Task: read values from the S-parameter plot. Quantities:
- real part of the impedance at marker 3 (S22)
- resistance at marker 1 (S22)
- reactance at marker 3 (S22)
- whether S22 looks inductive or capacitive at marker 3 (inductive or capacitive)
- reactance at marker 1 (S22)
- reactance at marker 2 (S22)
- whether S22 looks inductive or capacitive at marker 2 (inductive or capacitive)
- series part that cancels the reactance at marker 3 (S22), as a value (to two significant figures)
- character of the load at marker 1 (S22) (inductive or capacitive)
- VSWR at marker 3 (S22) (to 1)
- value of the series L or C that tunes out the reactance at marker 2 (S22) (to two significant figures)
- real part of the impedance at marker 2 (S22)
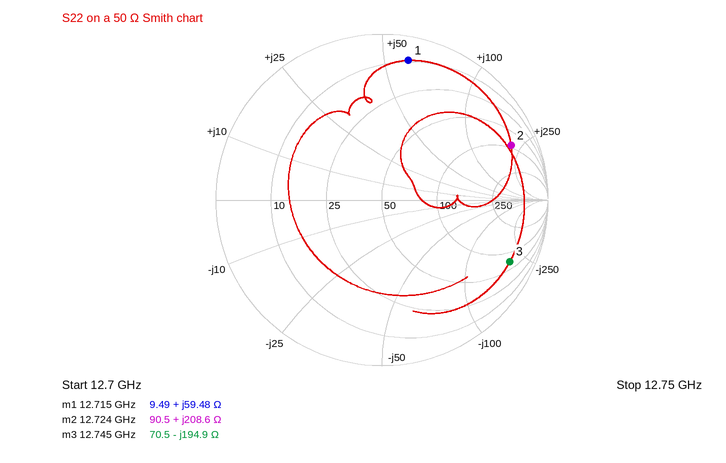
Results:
70.5 Ω
9.49 Ω
-194.9 Ω
capacitive
+59.48 Ω
+208.6 Ω
inductive
2.4 nH
inductive
13
60 fF
90.5 Ω
